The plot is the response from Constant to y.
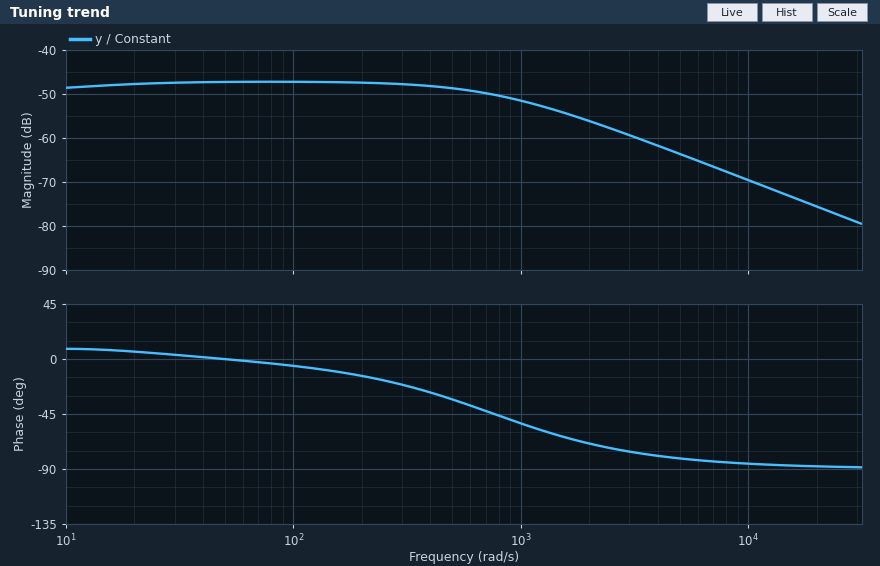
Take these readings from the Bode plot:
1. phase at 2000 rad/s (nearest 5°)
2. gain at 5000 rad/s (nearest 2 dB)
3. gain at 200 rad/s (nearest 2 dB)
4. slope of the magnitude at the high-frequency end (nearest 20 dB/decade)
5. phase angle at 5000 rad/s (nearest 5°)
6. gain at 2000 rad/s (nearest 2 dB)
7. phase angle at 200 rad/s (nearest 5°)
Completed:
-70°
-64 dB
-48 dB
-20 dB/decade
-80°
-56 dB
-15°
